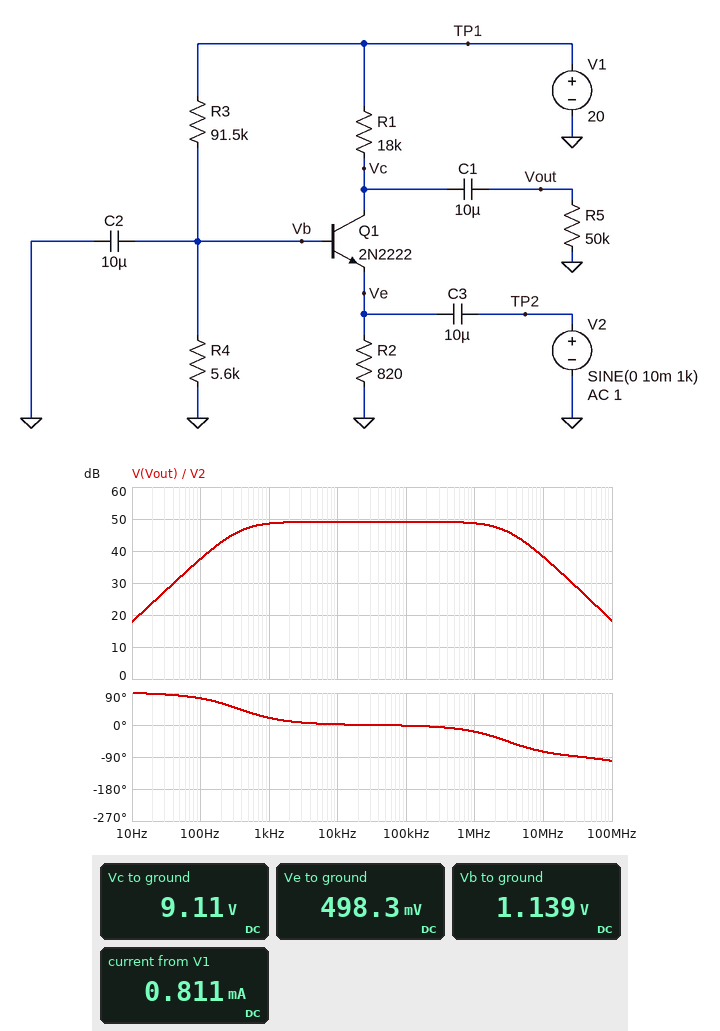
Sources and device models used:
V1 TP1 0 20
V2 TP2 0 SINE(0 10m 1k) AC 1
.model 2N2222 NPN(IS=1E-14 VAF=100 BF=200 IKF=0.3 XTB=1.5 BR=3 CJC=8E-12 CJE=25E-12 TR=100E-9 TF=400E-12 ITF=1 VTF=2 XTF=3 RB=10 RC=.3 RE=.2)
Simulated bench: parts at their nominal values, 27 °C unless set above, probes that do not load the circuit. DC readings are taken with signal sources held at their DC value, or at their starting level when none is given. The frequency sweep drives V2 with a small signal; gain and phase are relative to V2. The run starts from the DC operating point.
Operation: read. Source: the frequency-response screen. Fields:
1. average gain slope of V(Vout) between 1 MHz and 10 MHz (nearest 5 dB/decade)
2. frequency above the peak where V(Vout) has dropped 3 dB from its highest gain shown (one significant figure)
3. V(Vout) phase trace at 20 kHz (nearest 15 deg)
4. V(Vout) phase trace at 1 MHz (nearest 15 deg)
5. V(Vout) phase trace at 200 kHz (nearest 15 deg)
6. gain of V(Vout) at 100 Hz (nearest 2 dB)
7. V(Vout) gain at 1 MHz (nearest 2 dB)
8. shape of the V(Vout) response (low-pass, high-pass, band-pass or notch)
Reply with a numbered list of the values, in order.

1. -10 dB/decade
2. 3 MHz
3. 0 deg
4. -15 deg
5. 0 deg
6. 38 dB
7. 48 dB
8. band-pass
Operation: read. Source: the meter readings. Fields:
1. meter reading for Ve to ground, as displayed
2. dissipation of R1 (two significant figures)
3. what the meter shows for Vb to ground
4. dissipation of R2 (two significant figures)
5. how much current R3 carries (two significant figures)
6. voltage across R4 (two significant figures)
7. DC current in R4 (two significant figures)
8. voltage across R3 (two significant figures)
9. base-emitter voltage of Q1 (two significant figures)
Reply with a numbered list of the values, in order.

1. 498.3 mV
2. 6.6 mW
3. 1.139 V
4. 300 µW
5. 210 µA
6. 1.1 V
7. 200 µA
8. 19 V
9. 640 mV
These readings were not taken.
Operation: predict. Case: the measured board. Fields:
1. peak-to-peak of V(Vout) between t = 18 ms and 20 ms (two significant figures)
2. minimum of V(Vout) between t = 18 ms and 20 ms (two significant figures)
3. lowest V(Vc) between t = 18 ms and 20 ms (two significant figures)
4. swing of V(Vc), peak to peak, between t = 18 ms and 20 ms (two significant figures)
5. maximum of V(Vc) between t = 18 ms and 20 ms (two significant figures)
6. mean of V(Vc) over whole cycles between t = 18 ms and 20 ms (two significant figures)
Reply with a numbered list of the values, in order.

1. 5.3 V
2. -2.9 V
3. 6.2 V
4. 5.3 V
5. 12 V
6. 9.1 V
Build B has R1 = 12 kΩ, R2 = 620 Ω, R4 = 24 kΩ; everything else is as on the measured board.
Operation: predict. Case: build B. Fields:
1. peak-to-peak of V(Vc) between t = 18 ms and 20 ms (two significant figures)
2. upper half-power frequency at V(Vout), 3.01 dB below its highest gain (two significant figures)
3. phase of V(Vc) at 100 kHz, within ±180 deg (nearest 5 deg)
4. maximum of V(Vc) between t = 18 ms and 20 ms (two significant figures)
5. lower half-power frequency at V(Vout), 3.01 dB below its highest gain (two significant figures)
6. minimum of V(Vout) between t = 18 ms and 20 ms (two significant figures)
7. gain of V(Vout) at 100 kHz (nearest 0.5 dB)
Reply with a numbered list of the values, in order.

1. 690 mV
2. 1.4 MHz
3. -5 deg
4. 1.8 V
5. 540 Hz
6. -30 mV
7. 11.5 dB
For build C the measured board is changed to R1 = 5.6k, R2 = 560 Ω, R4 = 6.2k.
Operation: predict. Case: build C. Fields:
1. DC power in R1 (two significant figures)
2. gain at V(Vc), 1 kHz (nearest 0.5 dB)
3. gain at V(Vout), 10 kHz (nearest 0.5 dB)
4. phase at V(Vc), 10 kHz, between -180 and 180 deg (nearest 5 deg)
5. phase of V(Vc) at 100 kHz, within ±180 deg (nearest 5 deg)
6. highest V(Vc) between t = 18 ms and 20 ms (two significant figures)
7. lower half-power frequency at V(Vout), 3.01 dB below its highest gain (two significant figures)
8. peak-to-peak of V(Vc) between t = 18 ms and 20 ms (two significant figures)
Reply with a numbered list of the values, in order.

1. 6.1 mW
2. 44.0 dB
3. 45.5 dB
4. 5 deg
5. 0 deg
6. 16 V
7. 640 Hz
8. 3.2 V
